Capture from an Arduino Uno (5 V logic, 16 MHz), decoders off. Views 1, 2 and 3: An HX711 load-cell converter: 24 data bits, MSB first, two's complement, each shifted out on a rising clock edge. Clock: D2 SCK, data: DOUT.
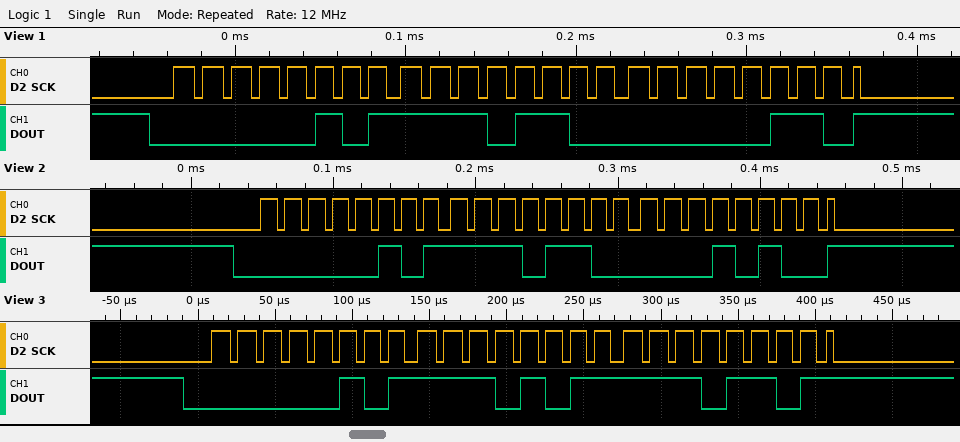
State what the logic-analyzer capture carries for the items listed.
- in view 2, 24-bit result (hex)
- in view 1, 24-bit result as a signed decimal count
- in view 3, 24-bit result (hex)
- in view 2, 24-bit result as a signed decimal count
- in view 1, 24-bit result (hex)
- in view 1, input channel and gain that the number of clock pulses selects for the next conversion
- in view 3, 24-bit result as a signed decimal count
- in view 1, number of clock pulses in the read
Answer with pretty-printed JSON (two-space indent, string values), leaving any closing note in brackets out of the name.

{
  "in view 2, 24-bit result": "0x05EC14",
  "in view 1, 24-bit result as a signed decimal count": "388102",
  "in view 3, 24-bit result": "0x05EBED",
  "in view 2, 24-bit result as a signed decimal count": "388116",
  "in view 1, 24-bit result": "0x05EC06",
  "in view 1, input channel and gain that the number of clock pulses selects for the next conversion": "channel A, gain 128",
  "in view 3, 24-bit result as a signed decimal count": "388077",
  "in view 1, number of clock pulses in the read": "25"
}
